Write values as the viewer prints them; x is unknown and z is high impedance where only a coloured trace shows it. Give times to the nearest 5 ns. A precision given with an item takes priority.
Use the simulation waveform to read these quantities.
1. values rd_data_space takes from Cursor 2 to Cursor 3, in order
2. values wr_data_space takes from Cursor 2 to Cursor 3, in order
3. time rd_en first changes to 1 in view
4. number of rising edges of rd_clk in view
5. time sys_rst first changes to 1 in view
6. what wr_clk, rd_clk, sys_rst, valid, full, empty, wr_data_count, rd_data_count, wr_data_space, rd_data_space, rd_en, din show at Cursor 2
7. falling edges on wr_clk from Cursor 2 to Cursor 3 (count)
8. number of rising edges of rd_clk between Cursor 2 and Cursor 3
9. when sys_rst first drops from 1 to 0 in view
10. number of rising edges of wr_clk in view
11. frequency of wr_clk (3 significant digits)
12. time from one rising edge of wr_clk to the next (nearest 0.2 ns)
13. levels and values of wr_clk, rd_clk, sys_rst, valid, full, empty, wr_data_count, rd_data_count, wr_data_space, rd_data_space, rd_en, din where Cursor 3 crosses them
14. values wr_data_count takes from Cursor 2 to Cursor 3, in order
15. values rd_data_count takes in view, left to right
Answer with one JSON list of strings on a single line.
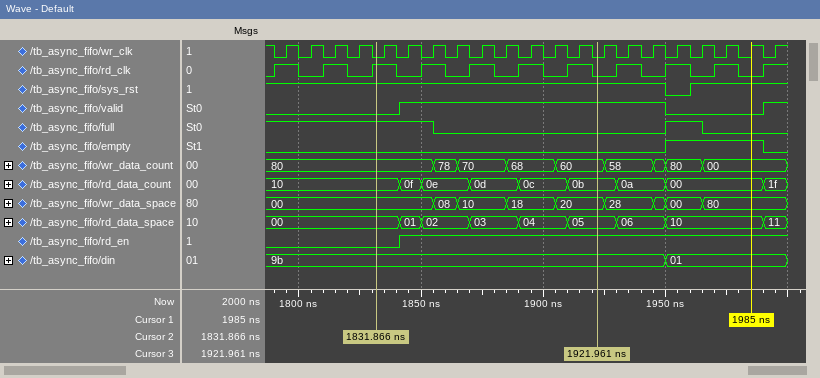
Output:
["00, 01, 02, 03, 04, 05", "00, 08, 10, 18, 20", "1840 ns", "11", "1960 ns", "wr_clk=0, rd_clk=1, sys_rst=1, valid=0, full=1, empty=0, wr_data_count=80, rd_data_count=10, wr_data_space=00, rd_data_space=00, rd_en=0, din=9b", "9", "4", "1950 ns", "21", "100 MHz", "10 ns", "wr_clk=0, rd_clk=0, sys_rst=1, valid=1, full=0, empty=0, wr_data_count=60, rd_data_count=0b, wr_data_space=20, rd_data_space=05, rd_en=1, din=9b", "80, 78, 70, 68, 60", "10, 0f, 0e, 0d, 0c, 0b, 0a, 00, 1f"]
